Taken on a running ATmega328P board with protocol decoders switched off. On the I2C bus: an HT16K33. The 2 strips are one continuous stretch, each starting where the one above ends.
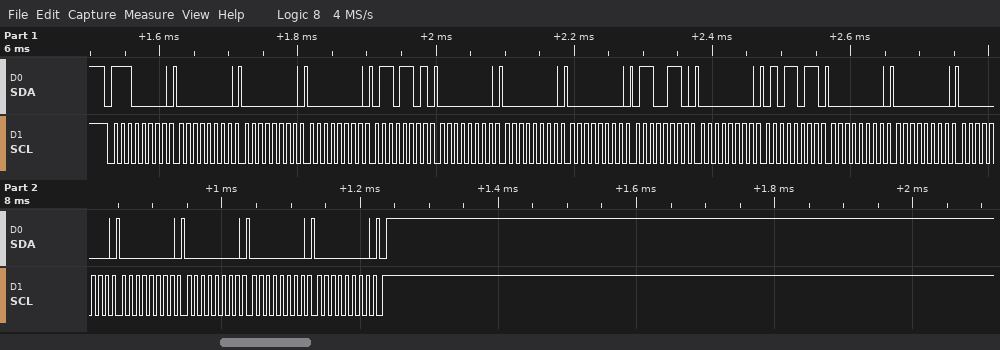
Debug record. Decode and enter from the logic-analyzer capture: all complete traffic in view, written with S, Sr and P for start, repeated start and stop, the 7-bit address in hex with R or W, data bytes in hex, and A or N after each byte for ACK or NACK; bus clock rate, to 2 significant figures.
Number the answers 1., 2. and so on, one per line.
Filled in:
1. S 70W A 00 A 00 A 00 A 6D A 00 A 00 A 00 A 66 A 00 A 5B A 00 A 00 A 00 A 00 A 00 A 00 A 00 A P
2. 100 kHz
